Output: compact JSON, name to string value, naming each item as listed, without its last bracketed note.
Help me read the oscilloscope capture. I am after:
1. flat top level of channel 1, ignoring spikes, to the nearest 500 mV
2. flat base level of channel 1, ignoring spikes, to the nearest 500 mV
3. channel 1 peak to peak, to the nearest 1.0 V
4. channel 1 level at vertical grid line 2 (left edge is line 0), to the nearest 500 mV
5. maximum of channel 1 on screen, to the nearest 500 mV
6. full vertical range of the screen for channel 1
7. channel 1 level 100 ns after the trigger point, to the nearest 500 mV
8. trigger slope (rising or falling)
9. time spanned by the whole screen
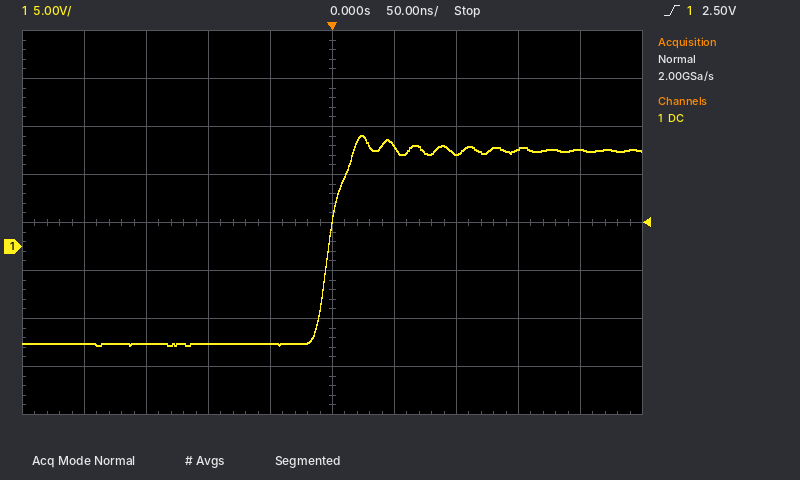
{"flat top level of channel 1, ignoring spikes, to the nearest 500 mV": "10.0 V", "flat base level of channel 1, ignoring spikes, to the nearest 500 mV": "-10.0 V", "channel 1 peak to peak, to the nearest 1.0 V": "22.0 V", "channel 1 level at vertical grid line 2 (left edge is line 0), to the nearest 500 mV": "-10.0 V", "maximum of channel 1 on screen, to the nearest 500 mV": "11.5 V", "full vertical range of the screen for channel 1": "40 V", "channel 1 level 100 ns after the trigger point, to the nearest 500 mV": "9.5 V", "trigger slope": "rising", "time spanned by the whole screen": "500 ns"}
